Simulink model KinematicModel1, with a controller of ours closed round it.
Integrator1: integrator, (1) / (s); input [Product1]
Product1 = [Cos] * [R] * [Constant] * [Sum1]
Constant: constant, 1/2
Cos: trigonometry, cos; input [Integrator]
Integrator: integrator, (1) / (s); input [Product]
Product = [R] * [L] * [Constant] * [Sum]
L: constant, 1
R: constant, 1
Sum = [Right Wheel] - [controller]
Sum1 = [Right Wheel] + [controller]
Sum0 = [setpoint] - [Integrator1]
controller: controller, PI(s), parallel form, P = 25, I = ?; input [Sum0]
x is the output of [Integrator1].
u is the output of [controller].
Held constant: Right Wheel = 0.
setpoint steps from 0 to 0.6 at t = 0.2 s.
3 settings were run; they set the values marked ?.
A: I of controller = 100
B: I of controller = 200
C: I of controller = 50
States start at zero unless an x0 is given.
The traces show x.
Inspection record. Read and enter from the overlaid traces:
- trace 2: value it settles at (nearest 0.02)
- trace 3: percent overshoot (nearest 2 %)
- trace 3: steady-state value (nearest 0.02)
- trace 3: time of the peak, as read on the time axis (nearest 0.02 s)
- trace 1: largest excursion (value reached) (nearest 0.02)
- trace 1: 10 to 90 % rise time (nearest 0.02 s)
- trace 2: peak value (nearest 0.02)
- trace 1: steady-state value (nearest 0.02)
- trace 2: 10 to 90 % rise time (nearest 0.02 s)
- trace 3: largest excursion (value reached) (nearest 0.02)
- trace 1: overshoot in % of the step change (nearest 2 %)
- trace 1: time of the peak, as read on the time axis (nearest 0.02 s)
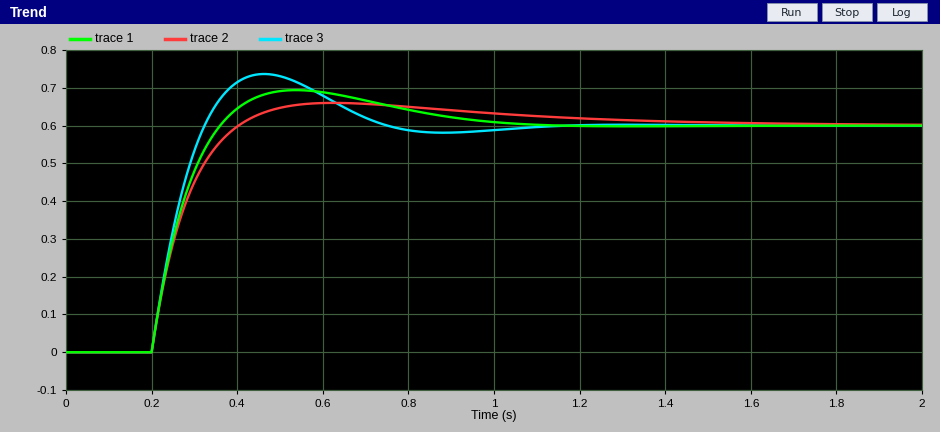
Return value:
0.60
22 %
0.60
0.46 s
0.70
0.12 s
0.66
0.60
0.14 s
0.74
16 %
0.54 s
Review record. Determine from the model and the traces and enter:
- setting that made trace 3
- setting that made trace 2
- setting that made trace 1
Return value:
B
C
A
